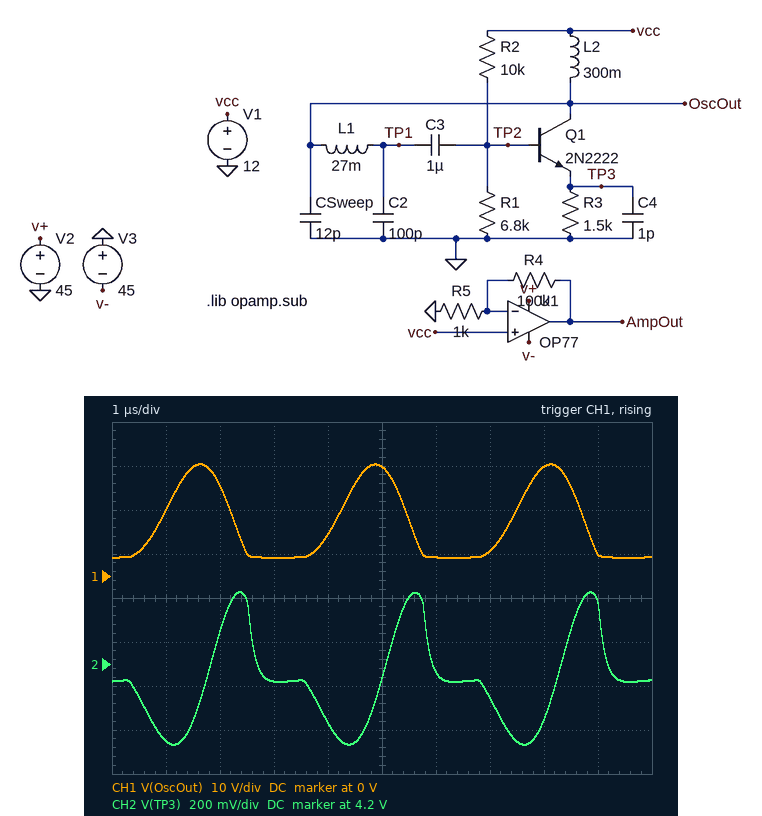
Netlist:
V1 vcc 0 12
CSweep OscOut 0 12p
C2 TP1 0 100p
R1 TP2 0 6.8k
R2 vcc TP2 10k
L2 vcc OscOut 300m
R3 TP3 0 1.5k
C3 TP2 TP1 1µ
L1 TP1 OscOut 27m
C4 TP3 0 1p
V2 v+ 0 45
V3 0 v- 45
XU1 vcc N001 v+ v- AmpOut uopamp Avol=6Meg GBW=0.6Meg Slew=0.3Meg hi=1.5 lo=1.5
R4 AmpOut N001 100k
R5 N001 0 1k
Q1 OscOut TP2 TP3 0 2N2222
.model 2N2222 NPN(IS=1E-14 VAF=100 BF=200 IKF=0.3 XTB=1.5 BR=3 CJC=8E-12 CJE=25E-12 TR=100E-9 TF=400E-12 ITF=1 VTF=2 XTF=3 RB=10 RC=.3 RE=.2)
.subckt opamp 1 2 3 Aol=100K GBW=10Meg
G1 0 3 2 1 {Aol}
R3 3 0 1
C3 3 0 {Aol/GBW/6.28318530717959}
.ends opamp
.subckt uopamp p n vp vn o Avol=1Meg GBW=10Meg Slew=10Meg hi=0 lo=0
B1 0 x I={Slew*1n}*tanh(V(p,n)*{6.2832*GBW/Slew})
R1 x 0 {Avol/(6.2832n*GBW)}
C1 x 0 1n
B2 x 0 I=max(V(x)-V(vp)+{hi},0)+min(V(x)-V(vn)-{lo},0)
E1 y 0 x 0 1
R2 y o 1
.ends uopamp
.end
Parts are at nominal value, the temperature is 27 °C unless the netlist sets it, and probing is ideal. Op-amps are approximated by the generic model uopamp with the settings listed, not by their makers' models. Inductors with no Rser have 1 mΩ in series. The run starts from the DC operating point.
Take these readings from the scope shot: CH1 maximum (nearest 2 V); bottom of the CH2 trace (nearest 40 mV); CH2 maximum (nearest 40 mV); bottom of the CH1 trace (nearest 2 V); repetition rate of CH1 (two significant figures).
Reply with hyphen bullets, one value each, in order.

- 26 V
- 3.84 V
- 4.52 V
- 4 V
- 310 kHz
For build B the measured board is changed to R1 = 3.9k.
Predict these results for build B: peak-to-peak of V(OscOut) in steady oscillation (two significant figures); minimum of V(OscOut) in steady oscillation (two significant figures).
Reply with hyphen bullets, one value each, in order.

- 24 V
- 2.7 V
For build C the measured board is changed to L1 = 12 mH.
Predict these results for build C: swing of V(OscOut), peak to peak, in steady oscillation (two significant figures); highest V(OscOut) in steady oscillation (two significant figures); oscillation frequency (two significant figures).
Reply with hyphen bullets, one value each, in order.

- 23 V
- 27 V
- 420 kHz
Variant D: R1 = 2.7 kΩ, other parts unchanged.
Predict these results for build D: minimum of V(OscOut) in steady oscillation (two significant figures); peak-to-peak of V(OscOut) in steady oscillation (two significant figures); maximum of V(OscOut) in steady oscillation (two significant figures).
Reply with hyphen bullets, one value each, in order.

- 1.9 V
- 25 V
- 27 V
